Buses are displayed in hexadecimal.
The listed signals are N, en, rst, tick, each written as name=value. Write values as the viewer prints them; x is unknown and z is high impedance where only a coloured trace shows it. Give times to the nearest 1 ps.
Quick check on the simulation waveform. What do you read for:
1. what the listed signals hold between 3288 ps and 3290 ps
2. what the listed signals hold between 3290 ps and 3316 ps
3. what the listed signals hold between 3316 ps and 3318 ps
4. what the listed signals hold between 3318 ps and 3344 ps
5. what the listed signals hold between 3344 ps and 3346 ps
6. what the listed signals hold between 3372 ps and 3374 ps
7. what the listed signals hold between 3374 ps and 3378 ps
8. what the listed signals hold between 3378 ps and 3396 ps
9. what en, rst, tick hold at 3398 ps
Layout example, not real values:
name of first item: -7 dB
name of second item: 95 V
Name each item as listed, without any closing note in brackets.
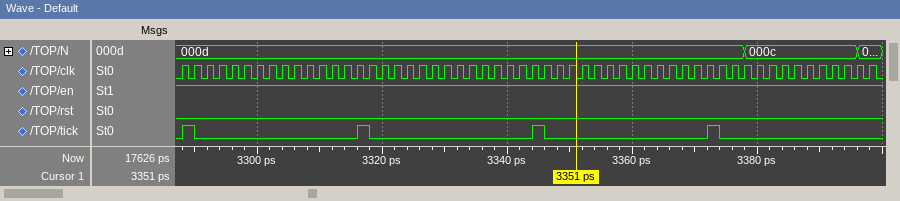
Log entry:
what the listed signals hold between 3288 ps and 3290 ps: N=000d, en=1, rst=0, tick=1
what the listed signals hold between 3290 ps and 3316 ps: N=000d, en=1, rst=0, tick=0
what the listed signals hold between 3316 ps and 3318 ps: N=000d, en=1, rst=0, tick=1
what the listed signals hold between 3318 ps and 3344 ps: N=000d, en=1, rst=0, tick=0
what the listed signals hold between 3344 ps and 3346 ps: N=000d, en=1, rst=0, tick=1
what the listed signals hold between 3372 ps and 3374 ps: N=000d, en=1, rst=0, tick=1
what the listed signals hold between 3374 ps and 3378 ps: N=000d, en=1, rst=0, tick=0
what the listed signals hold between 3378 ps and 3396 ps: N=000c, en=1, rst=0, tick=0
what en, rst, tick hold at 3398 ps: en=1, rst=0, tick=0
